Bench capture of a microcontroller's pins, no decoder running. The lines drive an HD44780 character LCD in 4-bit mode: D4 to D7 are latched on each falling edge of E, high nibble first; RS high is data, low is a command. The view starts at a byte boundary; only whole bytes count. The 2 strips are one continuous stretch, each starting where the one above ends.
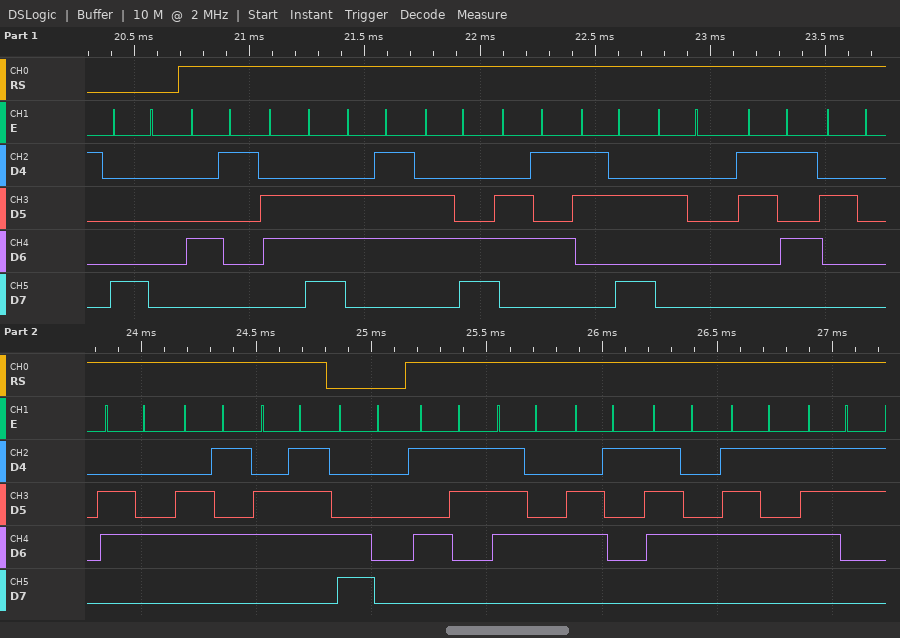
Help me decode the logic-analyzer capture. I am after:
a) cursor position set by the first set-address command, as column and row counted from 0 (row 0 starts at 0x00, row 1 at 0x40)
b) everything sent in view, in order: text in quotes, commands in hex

column 0, row 0
0x80 "Angle: 5 deg" 0xC0 "Status"
